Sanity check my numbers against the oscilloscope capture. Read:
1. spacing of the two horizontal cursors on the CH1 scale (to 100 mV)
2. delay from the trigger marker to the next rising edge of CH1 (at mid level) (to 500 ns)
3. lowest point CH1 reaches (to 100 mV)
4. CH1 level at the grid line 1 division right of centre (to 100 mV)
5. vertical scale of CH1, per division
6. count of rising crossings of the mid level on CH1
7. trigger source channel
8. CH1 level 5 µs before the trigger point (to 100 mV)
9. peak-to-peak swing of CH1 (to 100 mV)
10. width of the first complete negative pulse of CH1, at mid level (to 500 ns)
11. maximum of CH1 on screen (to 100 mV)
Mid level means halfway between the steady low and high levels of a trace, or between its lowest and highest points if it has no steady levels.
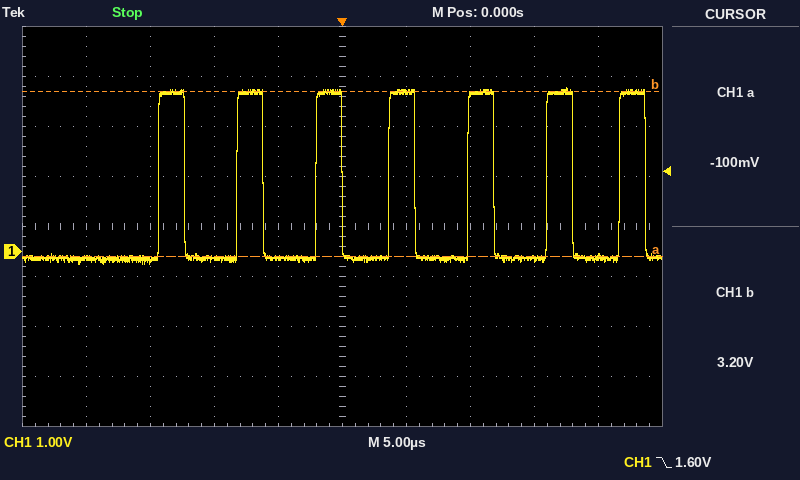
3.3 V
3.5 µs
-200 mV
3.2 V
1 V
7
CH1
-100 mV
3.5 V
4.0 µs
3.3 V
